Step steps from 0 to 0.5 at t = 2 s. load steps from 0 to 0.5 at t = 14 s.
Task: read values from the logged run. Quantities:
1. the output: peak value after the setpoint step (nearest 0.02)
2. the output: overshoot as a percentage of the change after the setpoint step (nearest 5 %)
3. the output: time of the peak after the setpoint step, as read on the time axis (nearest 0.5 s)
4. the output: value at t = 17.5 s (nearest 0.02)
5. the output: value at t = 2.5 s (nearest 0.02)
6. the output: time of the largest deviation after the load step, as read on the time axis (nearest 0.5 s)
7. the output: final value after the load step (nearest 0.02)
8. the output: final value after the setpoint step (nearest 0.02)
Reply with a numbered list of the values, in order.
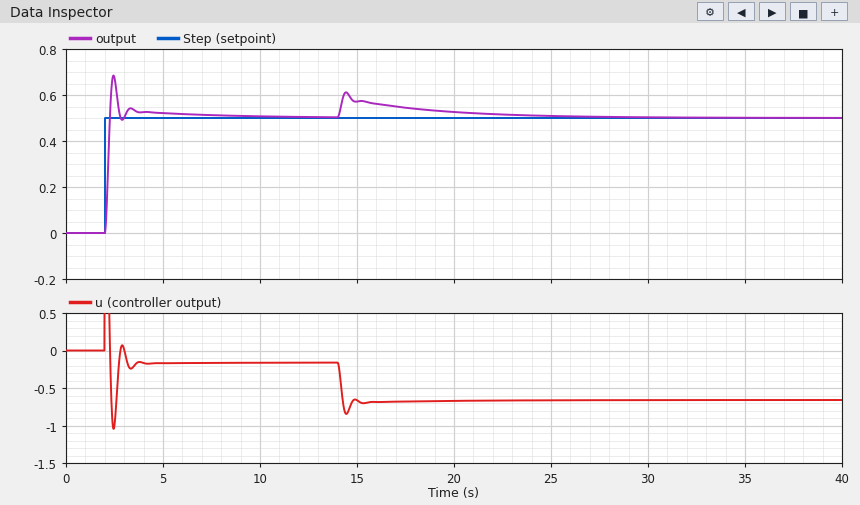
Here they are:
1. 0.68
2. 35 %
3. 2.5 s
4. 0.54
5. 0.68
6. 14.5 s
7. 0.50
8. 0.50
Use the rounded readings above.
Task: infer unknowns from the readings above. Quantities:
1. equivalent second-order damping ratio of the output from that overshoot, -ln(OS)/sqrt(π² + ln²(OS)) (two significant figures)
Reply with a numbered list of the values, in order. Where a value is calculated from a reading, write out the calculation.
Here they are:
1. ln(0.35) = -1.050; 1.050 / sqrt(9.870 + 1.102) = 0.32
